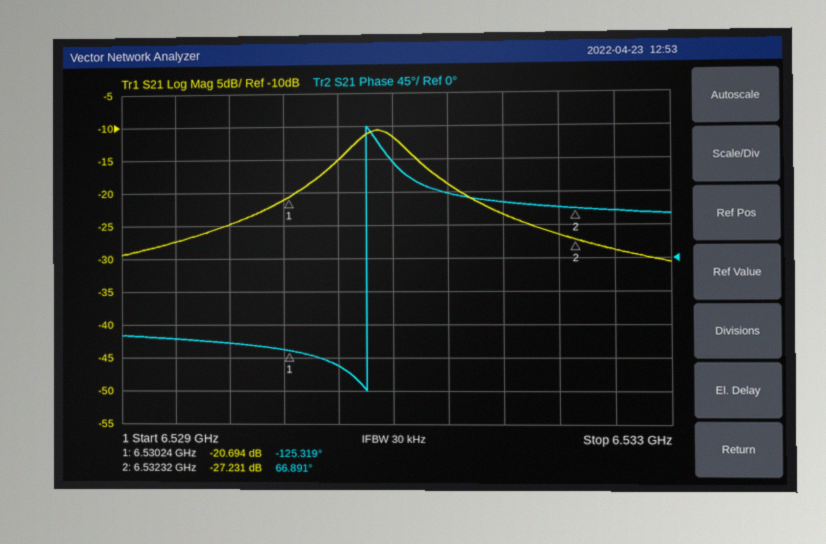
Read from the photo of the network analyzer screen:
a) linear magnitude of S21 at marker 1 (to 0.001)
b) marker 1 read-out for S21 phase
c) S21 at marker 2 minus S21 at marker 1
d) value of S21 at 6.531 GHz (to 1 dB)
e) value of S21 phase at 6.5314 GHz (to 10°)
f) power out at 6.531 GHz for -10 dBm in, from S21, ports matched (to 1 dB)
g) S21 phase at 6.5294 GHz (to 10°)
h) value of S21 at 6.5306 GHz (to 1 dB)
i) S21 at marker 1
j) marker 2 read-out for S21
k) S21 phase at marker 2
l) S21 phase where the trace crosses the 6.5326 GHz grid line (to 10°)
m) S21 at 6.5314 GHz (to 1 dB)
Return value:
0.092
-125.319°
-6.537 dB
-12 dB
90°
-22 dBm
-110°
-15 dB
-20.694 dB
-27.231 dB
66.891°
60°
-19 dB
